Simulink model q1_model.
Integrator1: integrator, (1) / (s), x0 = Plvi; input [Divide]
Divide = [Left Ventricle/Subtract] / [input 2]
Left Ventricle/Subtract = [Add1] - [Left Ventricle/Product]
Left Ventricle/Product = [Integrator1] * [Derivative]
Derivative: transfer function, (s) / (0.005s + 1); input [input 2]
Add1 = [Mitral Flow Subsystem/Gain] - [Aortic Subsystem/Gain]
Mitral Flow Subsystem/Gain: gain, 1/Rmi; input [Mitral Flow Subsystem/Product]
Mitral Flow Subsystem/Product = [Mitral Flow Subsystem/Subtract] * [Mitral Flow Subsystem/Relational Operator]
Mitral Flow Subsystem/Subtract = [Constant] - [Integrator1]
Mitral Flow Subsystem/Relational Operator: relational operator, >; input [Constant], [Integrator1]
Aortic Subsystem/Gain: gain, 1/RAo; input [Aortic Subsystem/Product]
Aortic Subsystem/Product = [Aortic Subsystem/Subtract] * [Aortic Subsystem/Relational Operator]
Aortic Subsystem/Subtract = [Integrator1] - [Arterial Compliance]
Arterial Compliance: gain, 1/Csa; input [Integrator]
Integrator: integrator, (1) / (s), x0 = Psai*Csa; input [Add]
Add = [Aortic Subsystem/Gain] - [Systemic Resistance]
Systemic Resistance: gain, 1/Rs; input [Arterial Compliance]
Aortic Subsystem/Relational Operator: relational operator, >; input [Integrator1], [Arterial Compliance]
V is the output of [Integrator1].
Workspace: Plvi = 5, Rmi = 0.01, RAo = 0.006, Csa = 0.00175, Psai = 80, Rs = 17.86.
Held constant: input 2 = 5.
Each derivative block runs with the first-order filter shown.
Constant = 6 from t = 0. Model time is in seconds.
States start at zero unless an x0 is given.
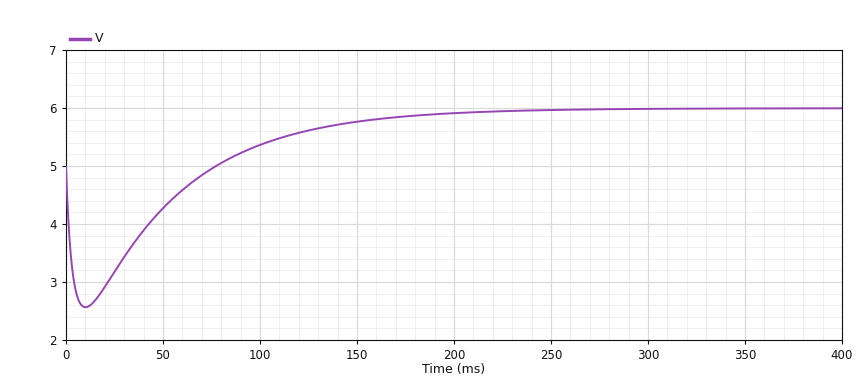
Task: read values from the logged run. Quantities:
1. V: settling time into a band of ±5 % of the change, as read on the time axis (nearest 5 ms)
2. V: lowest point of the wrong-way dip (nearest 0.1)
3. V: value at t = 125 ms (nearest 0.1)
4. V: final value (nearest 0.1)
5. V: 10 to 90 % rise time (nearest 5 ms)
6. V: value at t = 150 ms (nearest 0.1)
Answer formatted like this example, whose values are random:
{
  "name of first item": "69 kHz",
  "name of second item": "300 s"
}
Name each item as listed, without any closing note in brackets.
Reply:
{
  "V: settling time into a band of ±5 % of the change, as read on the time axis": "225 ms",
  "V: lowest point of the wrong-way dip": "2.6",
  "V: value at t = 125 ms": "5.6",
  "V: final value": "6.0",
  "V: 10 to 90 % rise time": "110 ms",
  "V: value at t = 150 ms": "5.8"
}
